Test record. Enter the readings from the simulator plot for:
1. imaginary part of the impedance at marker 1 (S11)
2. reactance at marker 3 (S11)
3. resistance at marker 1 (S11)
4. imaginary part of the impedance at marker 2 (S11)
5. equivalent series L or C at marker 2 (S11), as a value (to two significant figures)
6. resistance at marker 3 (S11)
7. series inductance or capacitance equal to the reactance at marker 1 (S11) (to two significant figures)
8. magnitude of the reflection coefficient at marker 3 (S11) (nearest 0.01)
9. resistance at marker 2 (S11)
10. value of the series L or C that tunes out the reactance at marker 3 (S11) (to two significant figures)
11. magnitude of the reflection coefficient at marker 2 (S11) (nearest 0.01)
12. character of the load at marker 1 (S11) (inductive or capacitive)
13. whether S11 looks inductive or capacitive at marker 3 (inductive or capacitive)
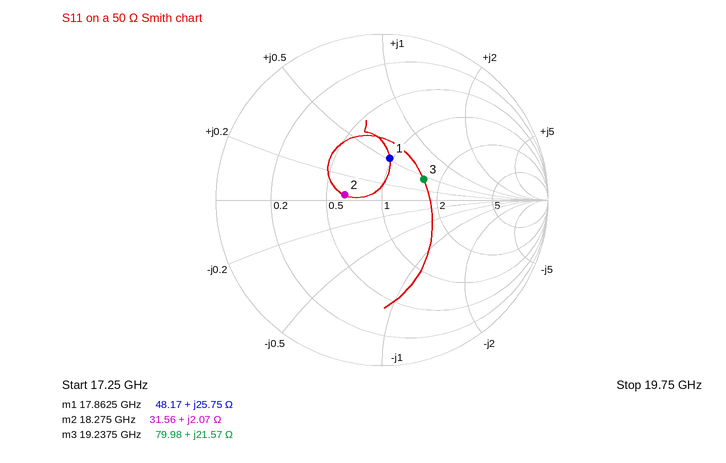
+25.75 Ω
+21.57 Ω
48.17 Ω
+2.07 Ω
18 pH
79.98 Ω
230 pH
0.28
31.56 Ω
380 fF
0.23
inductive
inductive
